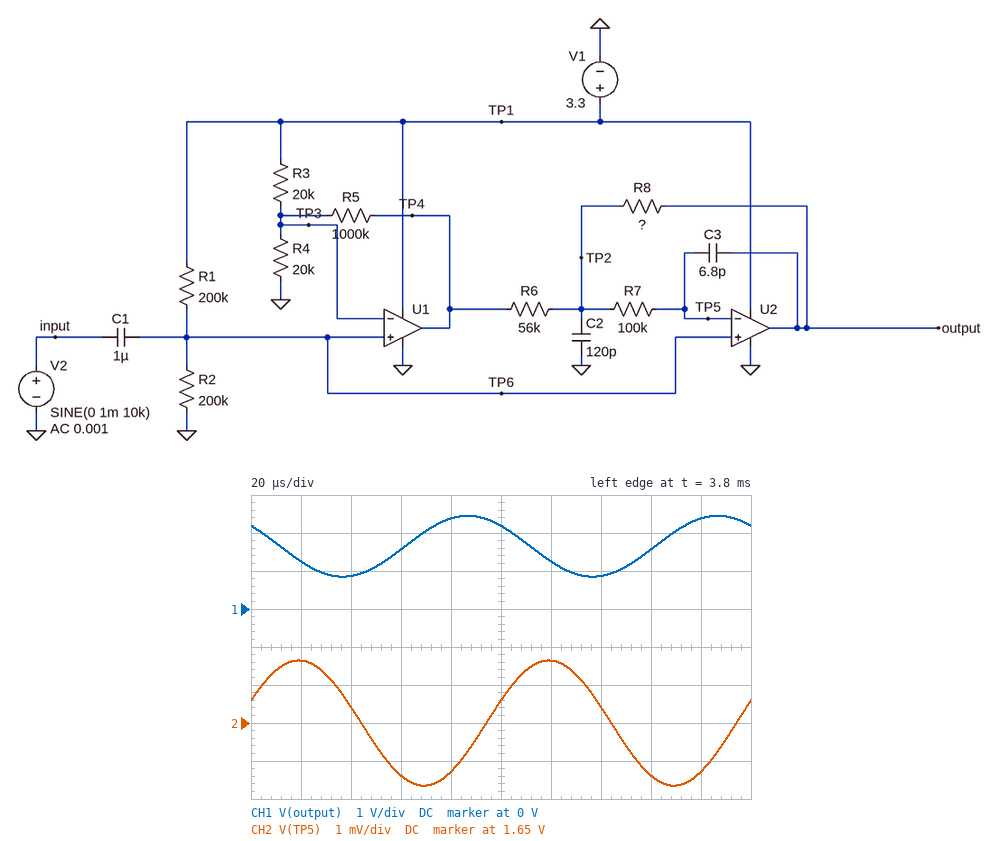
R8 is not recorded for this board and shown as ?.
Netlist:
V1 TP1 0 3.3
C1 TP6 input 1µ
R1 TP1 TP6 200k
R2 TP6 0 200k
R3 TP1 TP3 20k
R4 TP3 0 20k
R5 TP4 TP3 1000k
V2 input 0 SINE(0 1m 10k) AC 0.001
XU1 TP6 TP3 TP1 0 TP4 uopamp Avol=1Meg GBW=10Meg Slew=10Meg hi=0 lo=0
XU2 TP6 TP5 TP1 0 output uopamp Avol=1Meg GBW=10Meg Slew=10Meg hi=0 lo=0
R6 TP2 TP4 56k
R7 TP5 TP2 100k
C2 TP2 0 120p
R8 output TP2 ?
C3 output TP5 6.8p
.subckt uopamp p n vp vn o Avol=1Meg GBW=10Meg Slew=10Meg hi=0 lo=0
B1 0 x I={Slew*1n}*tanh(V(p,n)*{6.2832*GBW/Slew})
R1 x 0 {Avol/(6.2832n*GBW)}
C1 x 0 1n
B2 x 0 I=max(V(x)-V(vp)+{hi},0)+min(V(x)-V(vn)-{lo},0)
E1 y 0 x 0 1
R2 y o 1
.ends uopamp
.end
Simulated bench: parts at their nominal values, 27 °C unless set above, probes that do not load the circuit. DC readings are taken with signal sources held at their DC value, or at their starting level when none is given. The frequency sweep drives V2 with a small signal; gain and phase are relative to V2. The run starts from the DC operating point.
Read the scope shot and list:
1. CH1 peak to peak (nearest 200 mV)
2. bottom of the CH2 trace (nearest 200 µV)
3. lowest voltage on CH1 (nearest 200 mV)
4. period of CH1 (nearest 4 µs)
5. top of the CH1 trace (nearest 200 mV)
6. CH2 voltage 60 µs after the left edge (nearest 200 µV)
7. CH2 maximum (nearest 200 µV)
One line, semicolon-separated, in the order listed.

1.6 V; 1.6484 V; 800 mV; 100 µs; 2.4 V; 1.6486 V; 1.6516 V
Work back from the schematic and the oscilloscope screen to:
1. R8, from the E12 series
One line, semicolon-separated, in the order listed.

470 kΩ
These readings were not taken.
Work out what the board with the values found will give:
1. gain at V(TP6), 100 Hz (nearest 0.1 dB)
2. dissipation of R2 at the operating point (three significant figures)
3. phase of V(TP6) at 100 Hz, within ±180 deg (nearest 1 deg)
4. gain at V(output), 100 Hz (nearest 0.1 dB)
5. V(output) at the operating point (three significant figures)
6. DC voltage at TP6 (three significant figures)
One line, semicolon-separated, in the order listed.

0 dB; 13.6 µW; 1 deg; 58.5 dB; 1.65 V; 1.65 V
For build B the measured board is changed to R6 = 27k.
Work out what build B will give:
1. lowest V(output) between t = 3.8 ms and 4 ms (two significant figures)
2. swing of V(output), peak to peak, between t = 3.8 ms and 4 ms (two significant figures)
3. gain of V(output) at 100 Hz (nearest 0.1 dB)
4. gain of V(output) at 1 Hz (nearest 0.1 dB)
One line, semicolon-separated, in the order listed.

330 mV; 2.6 V; 64.8 dB; 59.3 dB
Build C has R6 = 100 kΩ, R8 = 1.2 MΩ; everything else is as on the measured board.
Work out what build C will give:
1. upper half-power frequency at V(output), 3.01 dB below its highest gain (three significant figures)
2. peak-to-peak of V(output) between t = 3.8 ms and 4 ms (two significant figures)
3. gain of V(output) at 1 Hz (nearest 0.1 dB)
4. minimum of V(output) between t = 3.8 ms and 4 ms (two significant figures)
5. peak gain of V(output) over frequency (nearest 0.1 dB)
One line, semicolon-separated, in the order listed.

12.5 kHz; 1.9 V; 56.1 dB; 690 mV; 61.6 dB
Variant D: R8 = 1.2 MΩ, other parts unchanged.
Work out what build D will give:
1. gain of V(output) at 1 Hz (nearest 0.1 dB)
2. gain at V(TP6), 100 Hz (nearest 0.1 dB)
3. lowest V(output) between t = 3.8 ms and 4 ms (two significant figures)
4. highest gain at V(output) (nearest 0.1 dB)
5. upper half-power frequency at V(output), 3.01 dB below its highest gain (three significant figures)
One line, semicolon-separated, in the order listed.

61.1 dB; 0 dB; 330 mV; 66.6 dB; 8.02 kHz
